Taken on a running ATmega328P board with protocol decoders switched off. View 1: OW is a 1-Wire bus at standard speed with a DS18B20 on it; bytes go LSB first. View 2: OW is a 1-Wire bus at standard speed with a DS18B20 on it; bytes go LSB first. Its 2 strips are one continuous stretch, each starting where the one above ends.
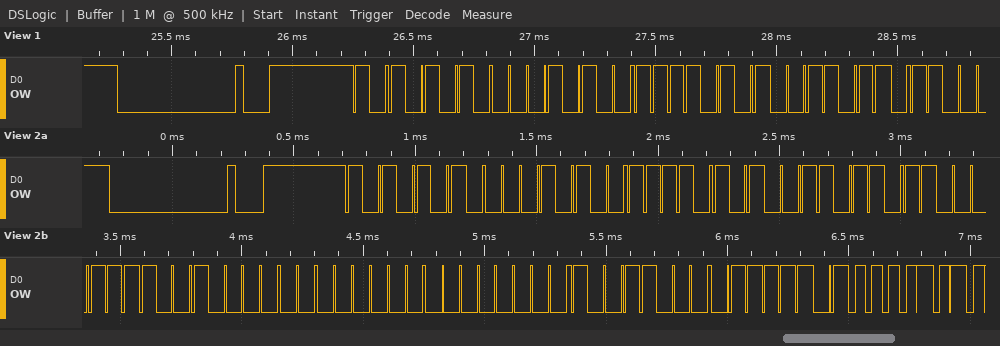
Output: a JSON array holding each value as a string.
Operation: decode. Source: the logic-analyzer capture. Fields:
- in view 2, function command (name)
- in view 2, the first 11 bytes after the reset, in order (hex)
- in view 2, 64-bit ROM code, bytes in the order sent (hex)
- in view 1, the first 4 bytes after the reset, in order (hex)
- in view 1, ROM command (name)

["Read Scratchpad", "55 28 AF 6C E3 09 00 00 19 BE 50", "28 AF 6C E3 09 00 00 19", "55 28 AF 6C", "Match ROM"]
